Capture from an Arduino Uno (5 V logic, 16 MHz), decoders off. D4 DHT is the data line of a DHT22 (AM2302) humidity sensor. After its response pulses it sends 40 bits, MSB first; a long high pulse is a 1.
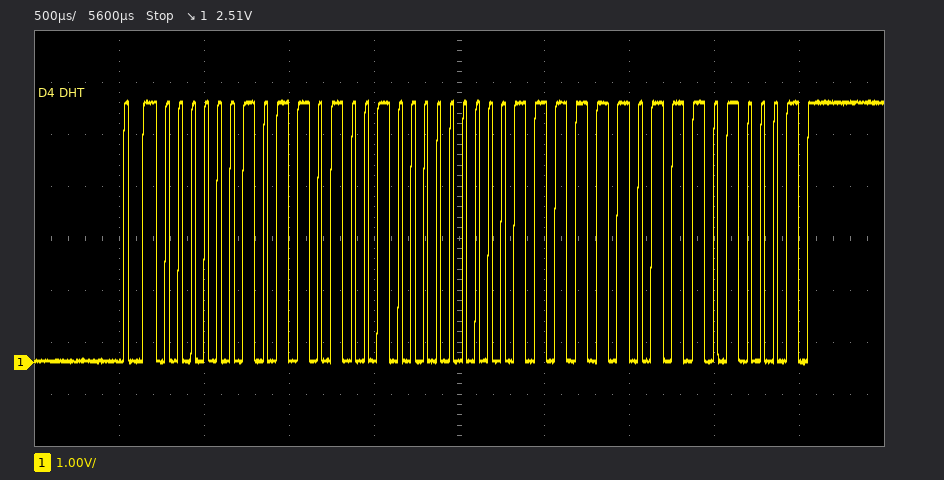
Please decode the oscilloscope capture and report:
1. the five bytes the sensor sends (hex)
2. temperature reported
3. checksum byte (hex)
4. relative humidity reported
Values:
02 D2 00 FD D1
25.3 °C
0xD1
72.2 %
